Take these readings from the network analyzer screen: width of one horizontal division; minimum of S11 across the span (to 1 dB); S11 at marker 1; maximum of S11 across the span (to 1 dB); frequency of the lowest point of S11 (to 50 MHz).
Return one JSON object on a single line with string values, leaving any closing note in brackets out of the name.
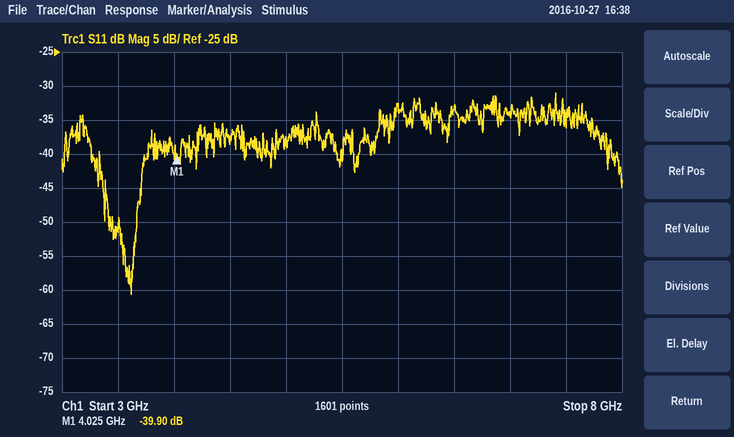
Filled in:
{"width of one horizontal division": "500 MHz", "minimum of S11 across the span": "-61 dB", "S11 at marker 1": "-39.90 dB", "maximum of S11 across the span": "-31 dB", "frequency of the lowest point of S11": "3.60 GHz"}
